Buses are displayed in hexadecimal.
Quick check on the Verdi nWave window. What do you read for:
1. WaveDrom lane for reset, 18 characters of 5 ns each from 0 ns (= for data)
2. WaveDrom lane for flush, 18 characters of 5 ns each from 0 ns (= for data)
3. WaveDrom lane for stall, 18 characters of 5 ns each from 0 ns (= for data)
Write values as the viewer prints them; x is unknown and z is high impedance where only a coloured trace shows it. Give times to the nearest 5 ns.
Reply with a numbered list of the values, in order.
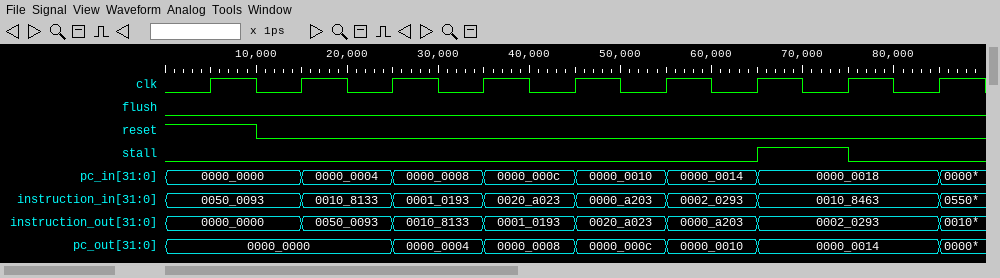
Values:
1. {name: 'reset', wave: '1.0...............'}
2. {name: 'flush', wave: '0.................'}
3. {name: 'stall', wave: '0............1.0..'}
